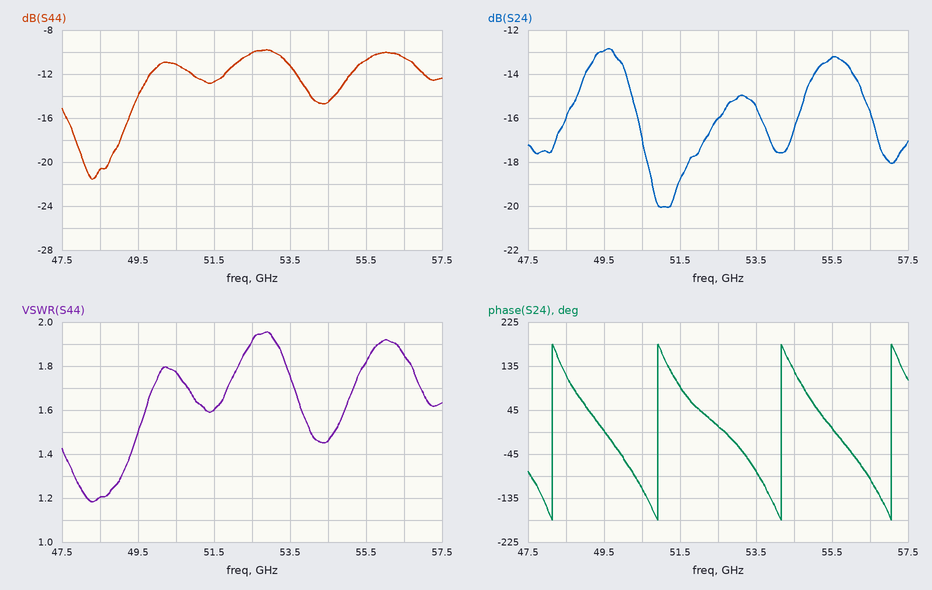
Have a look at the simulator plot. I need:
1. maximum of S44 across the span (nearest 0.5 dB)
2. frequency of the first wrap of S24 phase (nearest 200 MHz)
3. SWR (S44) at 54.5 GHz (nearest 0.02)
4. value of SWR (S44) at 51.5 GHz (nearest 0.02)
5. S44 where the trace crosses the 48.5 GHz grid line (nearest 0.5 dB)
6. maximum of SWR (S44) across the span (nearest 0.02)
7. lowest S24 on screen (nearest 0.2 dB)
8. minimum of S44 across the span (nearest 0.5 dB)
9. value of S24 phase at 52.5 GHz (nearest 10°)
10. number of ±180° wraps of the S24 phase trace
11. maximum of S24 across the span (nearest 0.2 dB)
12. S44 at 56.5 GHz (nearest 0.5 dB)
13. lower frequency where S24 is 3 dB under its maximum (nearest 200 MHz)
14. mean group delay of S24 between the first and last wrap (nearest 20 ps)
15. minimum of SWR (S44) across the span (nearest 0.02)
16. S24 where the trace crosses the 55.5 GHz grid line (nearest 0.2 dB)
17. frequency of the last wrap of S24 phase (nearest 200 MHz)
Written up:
-10.0 dB
48.2 GHz
1.46
1.60
-20.5 dB
1.96
-20.0 dB
-21.5 dB
10°
4
-12.8 dB
-10.5 dB
48.6 GHz
340 ps
1.18
-13.2 dB
57.0 GHz
